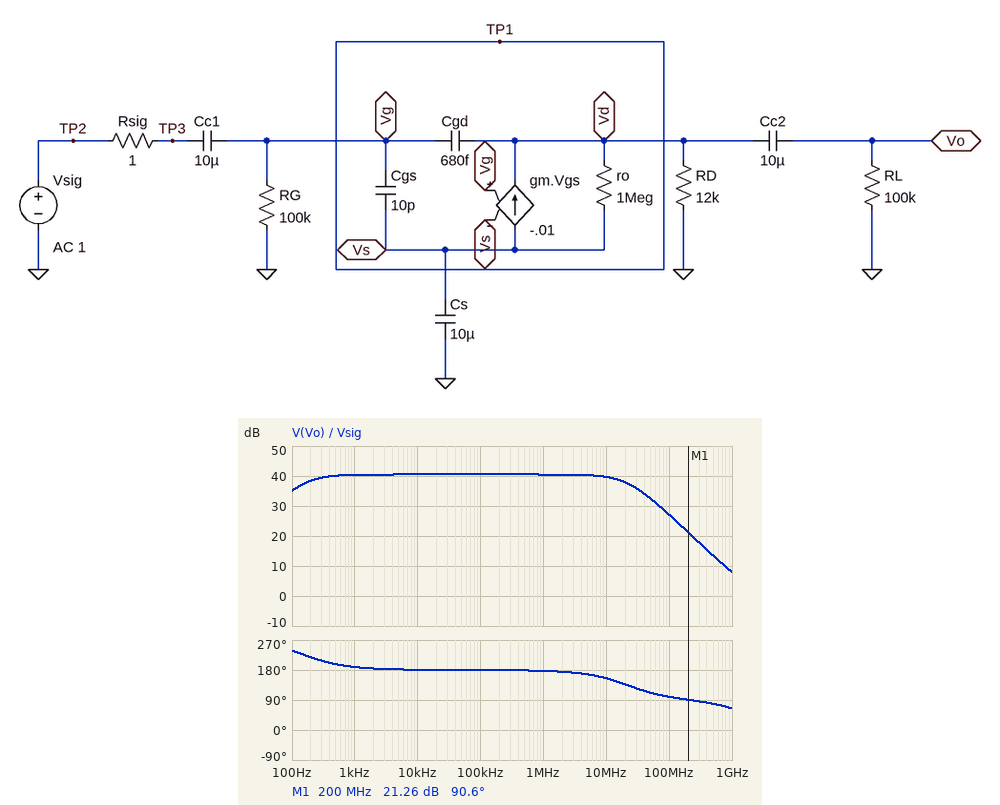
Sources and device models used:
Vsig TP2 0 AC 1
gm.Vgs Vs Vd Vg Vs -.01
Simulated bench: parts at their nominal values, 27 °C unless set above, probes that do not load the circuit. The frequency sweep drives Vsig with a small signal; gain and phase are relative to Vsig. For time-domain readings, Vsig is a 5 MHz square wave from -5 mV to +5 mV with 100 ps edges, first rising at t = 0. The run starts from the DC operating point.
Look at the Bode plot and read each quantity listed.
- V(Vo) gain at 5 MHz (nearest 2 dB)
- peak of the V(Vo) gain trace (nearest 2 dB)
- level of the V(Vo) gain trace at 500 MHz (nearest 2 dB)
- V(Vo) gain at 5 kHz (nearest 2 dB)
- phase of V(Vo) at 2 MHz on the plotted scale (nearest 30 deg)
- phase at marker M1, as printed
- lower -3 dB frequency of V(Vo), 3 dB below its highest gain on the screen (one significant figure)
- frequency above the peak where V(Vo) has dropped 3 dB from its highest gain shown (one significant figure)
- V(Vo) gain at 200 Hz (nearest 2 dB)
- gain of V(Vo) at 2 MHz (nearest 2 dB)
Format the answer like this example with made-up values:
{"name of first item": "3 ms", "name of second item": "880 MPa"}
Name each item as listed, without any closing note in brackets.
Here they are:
{"V(Vo) gain at 5 MHz": "40 dB", "peak of the V(Vo) gain trace": "40 dB", "level of the V(Vo) gain trace at 500 MHz": "14 dB", "V(Vo) gain at 5 kHz": "40 dB", "phase of V(Vo) at 2 MHz on the plotted scale": "180 deg", "phase at marker M1, as printed": "90.6 deg", "lower -3 dB frequency of V(Vo), 3 dB below its highest gain on the screen": "200 Hz", "frequency above the peak where V(Vo) has dropped 3 dB from its highest gain shown": "20 MHz", "V(Vo) gain at 200 Hz": "38 dB", "gain of V(Vo) at 2 MHz": "40 dB"}
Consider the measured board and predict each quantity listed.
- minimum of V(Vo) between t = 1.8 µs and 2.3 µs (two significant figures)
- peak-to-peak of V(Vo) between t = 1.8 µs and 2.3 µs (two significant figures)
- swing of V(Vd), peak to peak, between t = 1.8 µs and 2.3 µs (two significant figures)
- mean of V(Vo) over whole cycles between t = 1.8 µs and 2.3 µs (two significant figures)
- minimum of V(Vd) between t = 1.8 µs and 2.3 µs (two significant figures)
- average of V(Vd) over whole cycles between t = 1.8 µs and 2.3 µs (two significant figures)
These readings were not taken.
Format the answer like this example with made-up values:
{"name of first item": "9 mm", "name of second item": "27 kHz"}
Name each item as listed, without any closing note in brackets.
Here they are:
{"minimum of V(Vo) between t = 1.8 µs and 2.3 µs": "-1.1 V", "peak-to-peak of V(Vo) between t = 1.8 µs and 2.3 µs": "1.1 V", "swing of V(Vd), peak to peak, between t = 1.8 µs and 2.3 µs": "1.1 V", "mean of V(Vo) over whole cycles between t = 1.8 µs and 2.3 µs": "-530 mV", "minimum of V(Vd) between t = 1.8 µs and 2.3 µs": "-1.1 V", "average of V(Vd) over whole cycles between t = 1.8 µs and 2.3 µs": "-530 mV"}
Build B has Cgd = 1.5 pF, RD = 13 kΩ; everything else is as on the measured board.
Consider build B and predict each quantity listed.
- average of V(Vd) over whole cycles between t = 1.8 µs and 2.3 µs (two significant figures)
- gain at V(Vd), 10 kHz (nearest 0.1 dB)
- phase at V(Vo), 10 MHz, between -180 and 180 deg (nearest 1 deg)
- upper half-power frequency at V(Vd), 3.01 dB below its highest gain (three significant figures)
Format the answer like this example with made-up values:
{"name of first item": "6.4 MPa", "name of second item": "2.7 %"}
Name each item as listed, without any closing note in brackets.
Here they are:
{"average of V(Vd) over whole cycles between t = 1.8 µs and 2.3 µs": "-570 mV", "gain at V(Vd), 10 kHz": "41.1 dB", "phase at V(Vo), 10 MHz, between -180 and 180 deg": "132 deg", "upper half-power frequency at V(Vd), 3.01 dB below its highest gain": "9.24 MHz"}
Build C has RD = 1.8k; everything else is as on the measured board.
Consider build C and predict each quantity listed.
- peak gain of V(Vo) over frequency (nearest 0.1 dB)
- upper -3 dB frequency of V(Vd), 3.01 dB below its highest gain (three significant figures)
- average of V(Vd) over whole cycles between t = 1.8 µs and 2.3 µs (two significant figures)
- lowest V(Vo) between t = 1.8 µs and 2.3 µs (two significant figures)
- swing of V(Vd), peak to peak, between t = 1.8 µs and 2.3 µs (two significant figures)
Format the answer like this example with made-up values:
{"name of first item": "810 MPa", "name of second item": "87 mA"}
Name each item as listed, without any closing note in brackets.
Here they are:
{"peak gain of V(Vo) over frequency": "24.9 dB", "upper -3 dB frequency of V(Vd), 3.01 dB below its highest gain": "132 MHz", "average of V(Vd) over whole cycles between t = 1.8 µs and 2.3 µs": "-88 mV", "lowest V(Vo) between t = 1.8 µs and 2.3 µs": "-180 mV", "swing of V(Vd), peak to peak, between t = 1.8 µs and 2.3 µs": "180 mV"}
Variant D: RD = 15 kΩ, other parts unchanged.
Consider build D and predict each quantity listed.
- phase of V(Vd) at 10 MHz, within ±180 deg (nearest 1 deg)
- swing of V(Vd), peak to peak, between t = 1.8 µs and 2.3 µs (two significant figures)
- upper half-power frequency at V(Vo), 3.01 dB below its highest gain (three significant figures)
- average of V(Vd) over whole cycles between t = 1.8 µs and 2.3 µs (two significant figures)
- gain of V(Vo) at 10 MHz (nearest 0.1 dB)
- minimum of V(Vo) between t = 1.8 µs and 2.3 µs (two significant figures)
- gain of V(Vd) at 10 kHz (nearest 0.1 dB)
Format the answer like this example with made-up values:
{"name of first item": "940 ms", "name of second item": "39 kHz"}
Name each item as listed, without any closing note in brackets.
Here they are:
{"phase of V(Vd) at 10 MHz, within ±180 deg": "151 deg", "swing of V(Vd), peak to peak, between t = 1.8 µs and 2.3 µs": "1.3 V", "upper half-power frequency at V(Vo), 3.01 dB below its highest gain": "18.0 MHz", "average of V(Vd) over whole cycles between t = 1.8 µs and 2.3 µs": "-640 mV", "gain of V(Vo) at 10 MHz": "41.0 dB", "minimum of V(Vo) between t = 1.8 µs and 2.3 µs": "-1.3 V", "gain of V(Vd) at 10 kHz": "42.2 dB"}
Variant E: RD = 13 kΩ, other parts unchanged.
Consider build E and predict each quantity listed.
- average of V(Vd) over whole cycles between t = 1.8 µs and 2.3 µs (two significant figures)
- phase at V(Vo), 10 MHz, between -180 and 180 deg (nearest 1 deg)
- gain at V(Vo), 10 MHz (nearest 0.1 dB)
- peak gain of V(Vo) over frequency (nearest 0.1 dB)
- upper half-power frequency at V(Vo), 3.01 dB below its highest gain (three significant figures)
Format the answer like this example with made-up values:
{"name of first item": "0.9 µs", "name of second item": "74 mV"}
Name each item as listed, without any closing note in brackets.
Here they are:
{"average of V(Vd) over whole cycles between t = 1.8 µs and 2.3 µs": "-570 mV", "phase at V(Vo), 10 MHz, between -180 and 180 deg": "154 deg", "gain at V(Vo), 10 MHz": "40.2 dB", "peak gain of V(Vo) over frequency": "41.1 dB", "upper half-power frequency at V(Vo), 3.01 dB below its highest gain": "20.4 MHz"}
